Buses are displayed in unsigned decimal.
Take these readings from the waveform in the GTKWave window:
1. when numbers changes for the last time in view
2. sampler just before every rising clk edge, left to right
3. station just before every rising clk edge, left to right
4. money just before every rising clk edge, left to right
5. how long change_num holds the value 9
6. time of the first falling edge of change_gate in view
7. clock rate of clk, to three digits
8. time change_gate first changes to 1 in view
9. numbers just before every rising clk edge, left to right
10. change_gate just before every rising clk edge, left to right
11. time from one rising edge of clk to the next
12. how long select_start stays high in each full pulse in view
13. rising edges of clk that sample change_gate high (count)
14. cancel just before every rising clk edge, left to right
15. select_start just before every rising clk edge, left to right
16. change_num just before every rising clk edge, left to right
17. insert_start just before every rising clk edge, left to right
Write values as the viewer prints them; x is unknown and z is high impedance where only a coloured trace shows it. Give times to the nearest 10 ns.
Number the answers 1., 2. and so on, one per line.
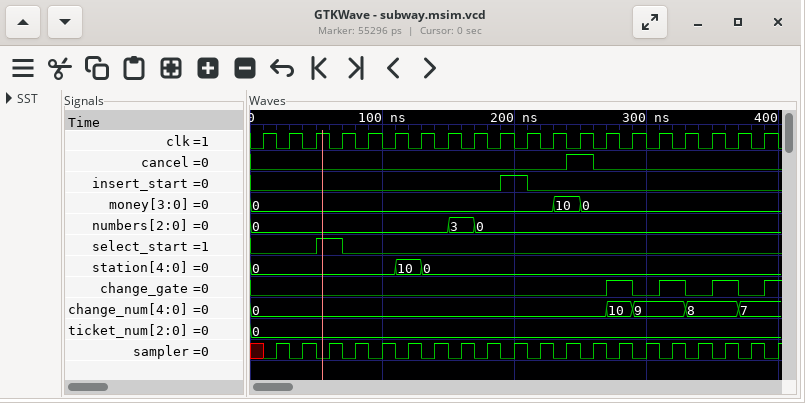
1. 170 ns
2. x 1 1 1 1 1 1 1 1 1 1 1 1 1 1 1 1 1 1 1
3. 0, 0, 0, 0, 0, 0, 10, 0, 0, 0, 0, 0, 0, 0, 0, 0, 0, 0, 0, 0
4. 0, 0, 0, 0, 0, 0, 0, 0, 0, 0, 0, 0, 10, 0, 0, 0, 0, 0, 0, 0
5. 40 ns
6. 290 ns
7. 50.0 MHz
8. 270 ns
9. 0, 0, 0, 0, 0, 0, 0, 0, 3, 0, 0, 0, 0, 0, 0, 0, 0, 0, 0, 0
10. 0 0 0 0 0 0 0 0 0 0 0 0 0 0 1 0 1 0 1 0
11. 20 ns
12. 20 ns
13. 3
14. 0 0 0 0 0 0 0 0 0 0 0 0 1 0 0 0 0 0 0 0
15. 0 0 0 1 0 0 0 0 0 0 0 0 0 0 0 0 0 0 0 0
16. 0, 0, 0, 0, 0, 0, 0, 0, 0, 0, 0, 0, 0, 0, 10, 9, 9, 8, 8, 7
17. 0 0 0 0 0 0 0 0 0 0 1 0 0 0 0 0 0 0 0 0
